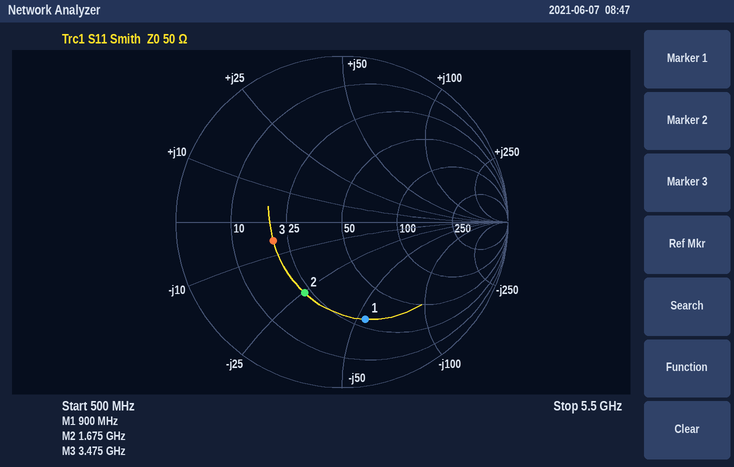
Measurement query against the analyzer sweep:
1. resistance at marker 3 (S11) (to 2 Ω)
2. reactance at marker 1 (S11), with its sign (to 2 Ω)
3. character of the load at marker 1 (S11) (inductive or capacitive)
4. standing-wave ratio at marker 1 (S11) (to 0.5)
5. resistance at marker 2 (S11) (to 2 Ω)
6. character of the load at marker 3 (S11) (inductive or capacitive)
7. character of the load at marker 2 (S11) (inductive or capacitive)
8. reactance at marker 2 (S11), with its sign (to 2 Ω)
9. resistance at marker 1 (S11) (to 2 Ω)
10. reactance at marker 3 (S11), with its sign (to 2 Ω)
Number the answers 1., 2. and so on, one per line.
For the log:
1. 20 Ω
2. -54 Ω
3. capacitive
4. 4.0
5. 22 Ω
6. capacitive
7. capacitive
8. -26 Ω
9. 30 Ω
10. -6 Ω
